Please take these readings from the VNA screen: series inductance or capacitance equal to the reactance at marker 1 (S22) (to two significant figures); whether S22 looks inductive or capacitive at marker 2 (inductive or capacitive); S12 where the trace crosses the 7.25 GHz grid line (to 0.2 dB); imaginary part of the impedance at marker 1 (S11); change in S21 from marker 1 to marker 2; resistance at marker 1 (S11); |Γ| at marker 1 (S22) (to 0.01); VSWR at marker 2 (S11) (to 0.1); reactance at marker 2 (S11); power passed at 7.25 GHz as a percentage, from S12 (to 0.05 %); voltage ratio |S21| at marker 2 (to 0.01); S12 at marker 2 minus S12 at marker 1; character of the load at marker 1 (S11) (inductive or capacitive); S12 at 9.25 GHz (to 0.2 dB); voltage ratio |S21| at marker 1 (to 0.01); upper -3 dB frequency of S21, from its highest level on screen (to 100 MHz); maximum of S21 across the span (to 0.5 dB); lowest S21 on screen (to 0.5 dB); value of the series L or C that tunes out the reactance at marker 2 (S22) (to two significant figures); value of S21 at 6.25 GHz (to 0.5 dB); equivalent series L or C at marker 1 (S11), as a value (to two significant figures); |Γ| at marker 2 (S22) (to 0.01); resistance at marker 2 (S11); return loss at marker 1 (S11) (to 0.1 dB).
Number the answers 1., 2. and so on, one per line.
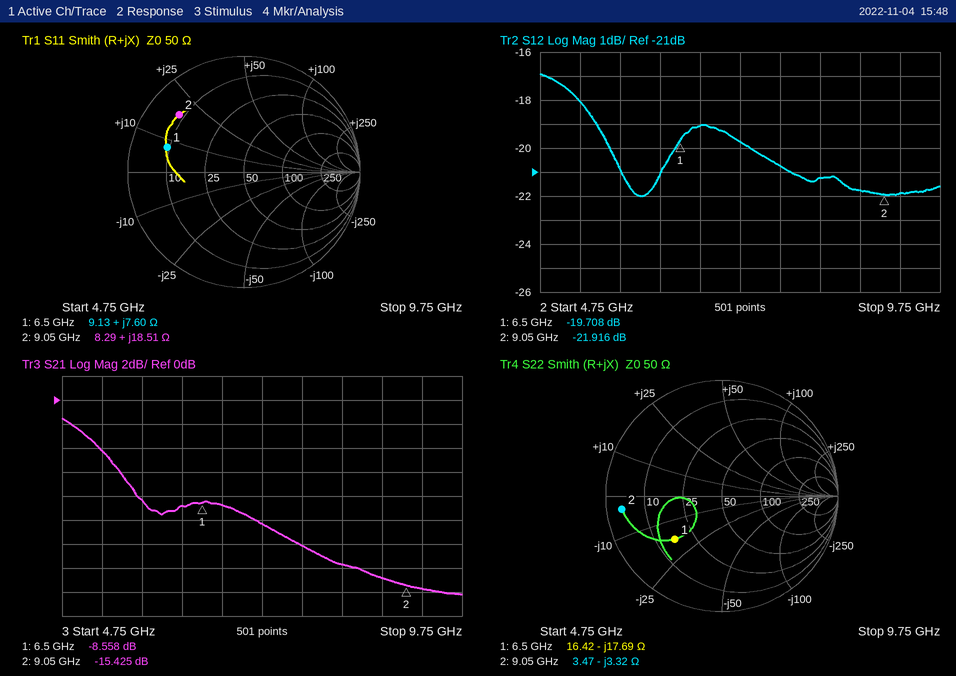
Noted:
1. 1.4 pF
2. capacitive
3. -19.8 dB
4. +7.60 Ω
5. -6.867 dB
6. 9.13 Ω
7. 0.55
8. 6.9
9. +18.51 Ω
10. 1.05 %
11. 0.17
12. -2.208 dB
13. inductive
14. -21.8 dB
15. 0.37
16. 5.3 GHz
17. -1.5 dB
18. -16.0 dB
19. 58 pH
20. -9.0 dB
21. 190 pH
22. 0.87
23. 8.29 Ω
24. 3.1 dB
